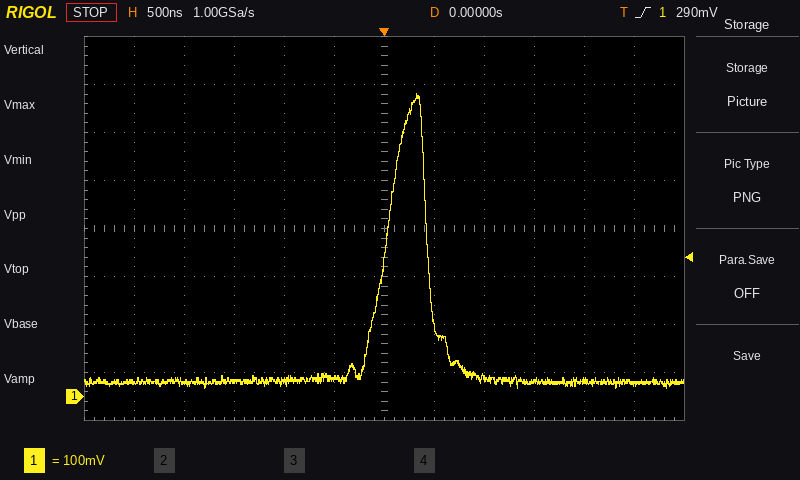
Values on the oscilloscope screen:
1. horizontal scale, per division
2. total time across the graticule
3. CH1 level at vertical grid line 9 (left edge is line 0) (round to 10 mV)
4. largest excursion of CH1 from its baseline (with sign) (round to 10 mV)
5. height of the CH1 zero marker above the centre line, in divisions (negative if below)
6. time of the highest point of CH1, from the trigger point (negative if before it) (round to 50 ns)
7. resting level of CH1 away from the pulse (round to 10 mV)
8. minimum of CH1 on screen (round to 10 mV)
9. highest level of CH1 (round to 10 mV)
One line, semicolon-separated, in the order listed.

500 ns; 6 µs; 30 mV; +600 mV; -3.5 div; +350 ns; 30 mV; 20 mV; 630 mV
